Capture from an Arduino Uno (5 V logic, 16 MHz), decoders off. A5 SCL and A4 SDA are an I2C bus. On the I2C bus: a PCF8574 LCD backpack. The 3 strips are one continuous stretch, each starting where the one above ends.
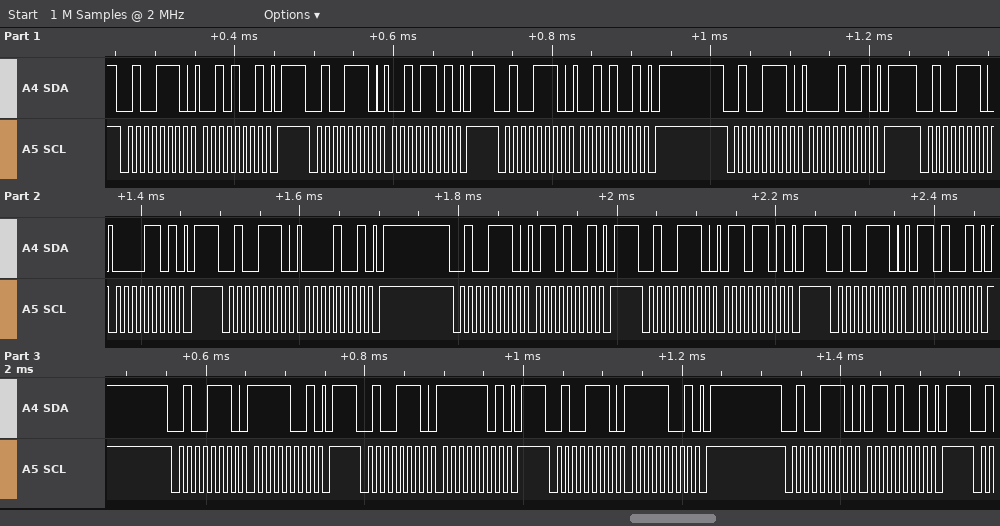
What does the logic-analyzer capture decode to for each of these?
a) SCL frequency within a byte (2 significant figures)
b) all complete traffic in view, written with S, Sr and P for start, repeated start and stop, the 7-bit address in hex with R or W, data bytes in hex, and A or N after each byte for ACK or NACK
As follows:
100 kHz
S 27W A 29 A P S 27W A 2D A P S 27W A 29 A P S 27W A 09 A P S 27W A 0D A P S 27W A 09 A P S 27W A 69 A P S 27W A 6D A P S 27W A 69 A P S 27W A F9 A P S 27W A FD A P S 27W A F9 A P S 27W A 69 A P
